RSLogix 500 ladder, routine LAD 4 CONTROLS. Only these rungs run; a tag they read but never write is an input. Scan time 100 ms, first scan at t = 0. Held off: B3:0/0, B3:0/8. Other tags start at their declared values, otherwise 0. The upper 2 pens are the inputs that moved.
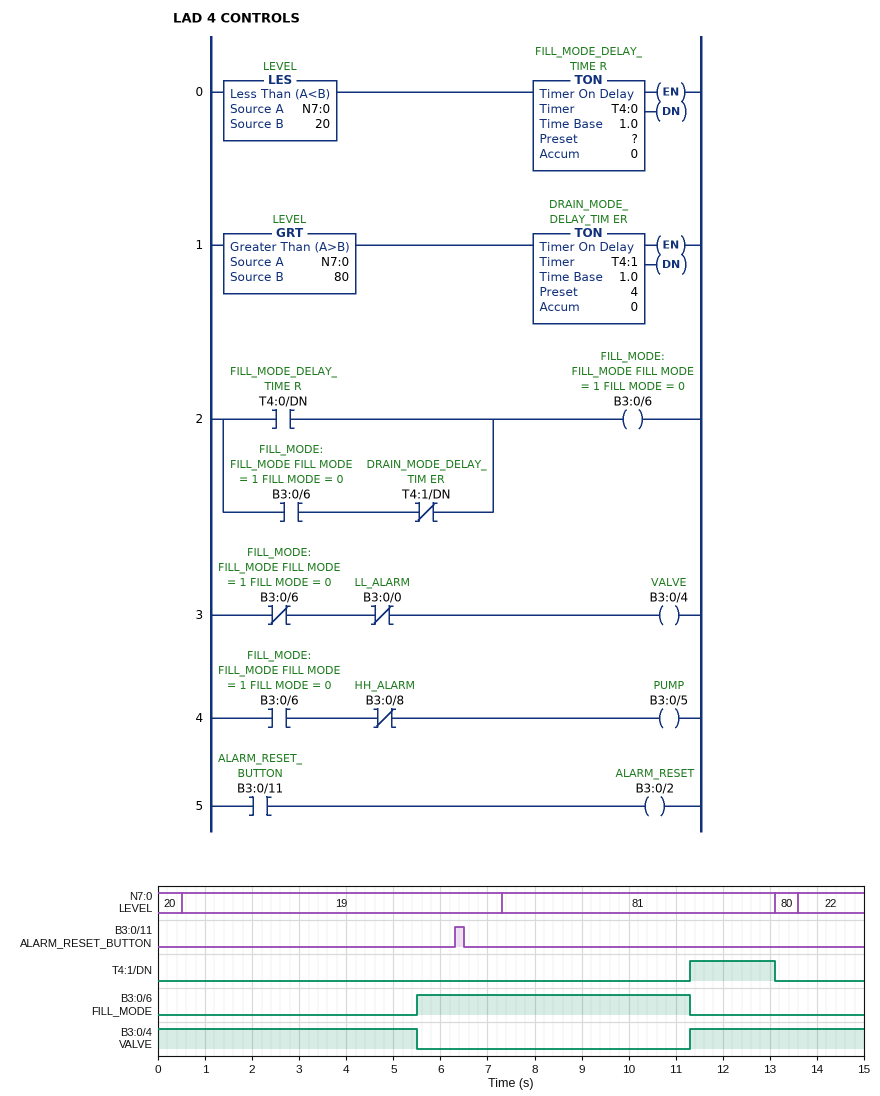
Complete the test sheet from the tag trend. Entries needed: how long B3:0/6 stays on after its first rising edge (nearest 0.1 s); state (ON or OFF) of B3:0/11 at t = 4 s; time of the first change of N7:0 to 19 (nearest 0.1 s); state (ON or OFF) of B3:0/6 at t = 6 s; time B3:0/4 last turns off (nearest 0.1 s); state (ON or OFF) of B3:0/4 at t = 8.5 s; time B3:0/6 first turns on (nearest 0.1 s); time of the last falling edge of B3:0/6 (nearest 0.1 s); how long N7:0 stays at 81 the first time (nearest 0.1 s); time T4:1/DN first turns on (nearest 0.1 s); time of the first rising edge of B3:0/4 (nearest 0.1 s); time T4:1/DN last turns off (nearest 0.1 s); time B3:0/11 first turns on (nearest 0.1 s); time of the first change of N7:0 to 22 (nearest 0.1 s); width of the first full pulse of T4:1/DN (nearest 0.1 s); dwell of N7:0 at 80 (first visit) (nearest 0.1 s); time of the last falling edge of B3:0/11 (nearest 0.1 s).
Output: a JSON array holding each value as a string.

["5.8 s", "OFF", "0.5 s", "ON", "5.5 s", "OFF", "5.5 s", "11.3 s", "5.8 s", "11.3 s", "11.3 s", "13.1 s", "6.3 s", "13.6 s", "1.8 s", "0.5 s", "6.5 s"]
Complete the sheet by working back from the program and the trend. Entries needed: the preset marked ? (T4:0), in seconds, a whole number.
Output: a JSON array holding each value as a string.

["5 s"]
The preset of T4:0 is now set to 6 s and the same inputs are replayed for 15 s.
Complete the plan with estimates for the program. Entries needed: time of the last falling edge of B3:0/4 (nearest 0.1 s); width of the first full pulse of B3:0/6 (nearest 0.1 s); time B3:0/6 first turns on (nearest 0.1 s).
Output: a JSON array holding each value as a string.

["6.5 s", "4.8 s", "6.5 s"]
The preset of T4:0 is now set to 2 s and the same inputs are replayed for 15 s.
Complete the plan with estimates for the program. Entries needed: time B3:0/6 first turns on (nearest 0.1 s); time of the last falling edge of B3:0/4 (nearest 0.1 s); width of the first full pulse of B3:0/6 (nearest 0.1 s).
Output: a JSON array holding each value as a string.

["2.5 s", "2.5 s", "8.8 s"]
